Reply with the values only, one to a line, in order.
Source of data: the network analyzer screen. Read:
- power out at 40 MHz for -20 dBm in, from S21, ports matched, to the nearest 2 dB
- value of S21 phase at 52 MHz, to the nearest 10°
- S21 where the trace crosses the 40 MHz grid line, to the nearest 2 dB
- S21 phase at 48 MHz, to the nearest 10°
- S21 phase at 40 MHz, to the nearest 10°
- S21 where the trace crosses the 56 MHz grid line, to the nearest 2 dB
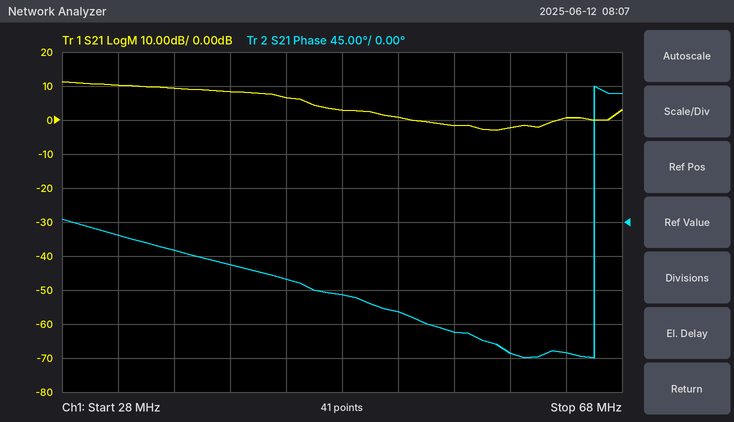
-12 dBm
-120°
8 dB
-100°
-60°
-2 dB
